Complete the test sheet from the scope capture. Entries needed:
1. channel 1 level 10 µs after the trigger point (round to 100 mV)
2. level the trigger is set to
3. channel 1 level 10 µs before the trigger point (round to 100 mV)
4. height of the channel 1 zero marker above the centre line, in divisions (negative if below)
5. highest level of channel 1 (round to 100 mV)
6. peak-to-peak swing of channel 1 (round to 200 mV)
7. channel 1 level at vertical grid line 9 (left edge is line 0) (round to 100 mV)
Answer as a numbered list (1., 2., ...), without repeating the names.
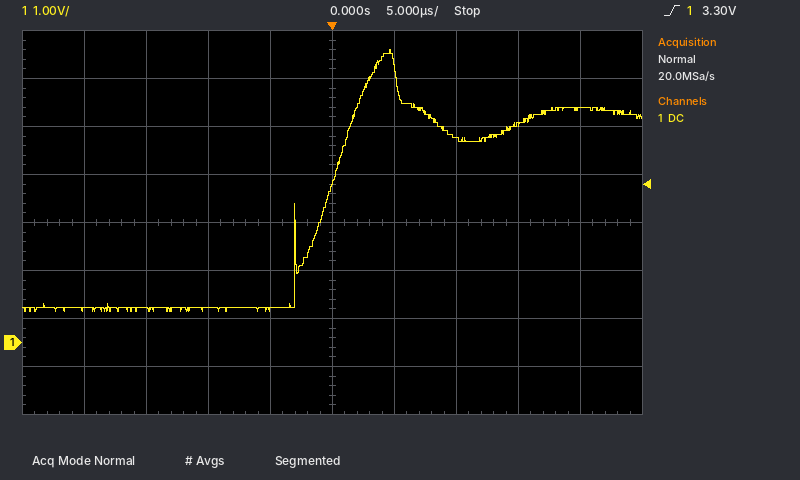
1. 4.2 V
2. 3.30 V
3. 700 mV
4. -2.5 div
5. 6.1 V
6. 5.4 V
7. 4.9 V
